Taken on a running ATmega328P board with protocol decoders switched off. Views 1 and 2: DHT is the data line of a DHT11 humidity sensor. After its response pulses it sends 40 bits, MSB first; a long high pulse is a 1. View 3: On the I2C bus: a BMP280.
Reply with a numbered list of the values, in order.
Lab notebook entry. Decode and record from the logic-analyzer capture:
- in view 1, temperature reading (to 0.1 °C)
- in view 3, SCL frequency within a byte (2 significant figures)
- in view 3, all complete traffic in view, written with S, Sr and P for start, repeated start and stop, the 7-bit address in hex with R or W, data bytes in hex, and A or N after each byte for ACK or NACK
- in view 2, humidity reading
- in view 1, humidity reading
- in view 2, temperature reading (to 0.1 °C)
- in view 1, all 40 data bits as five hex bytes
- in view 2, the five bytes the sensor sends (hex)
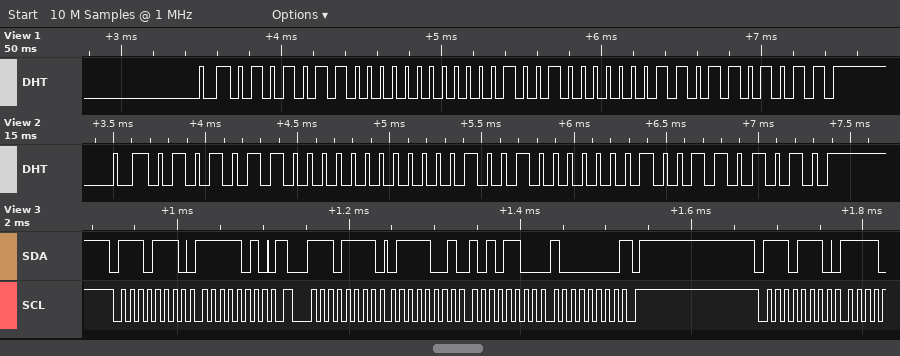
1. 18.3 °C
2. 100 kHz
3. S 77W A FA A Sr 77R A 79 A AC A 80 N P S 77W A
4. 86 %
5. 86 %
6. 18.2 °C
7. 56 00 12 03 6B
8. 56 00 12 02 6A
